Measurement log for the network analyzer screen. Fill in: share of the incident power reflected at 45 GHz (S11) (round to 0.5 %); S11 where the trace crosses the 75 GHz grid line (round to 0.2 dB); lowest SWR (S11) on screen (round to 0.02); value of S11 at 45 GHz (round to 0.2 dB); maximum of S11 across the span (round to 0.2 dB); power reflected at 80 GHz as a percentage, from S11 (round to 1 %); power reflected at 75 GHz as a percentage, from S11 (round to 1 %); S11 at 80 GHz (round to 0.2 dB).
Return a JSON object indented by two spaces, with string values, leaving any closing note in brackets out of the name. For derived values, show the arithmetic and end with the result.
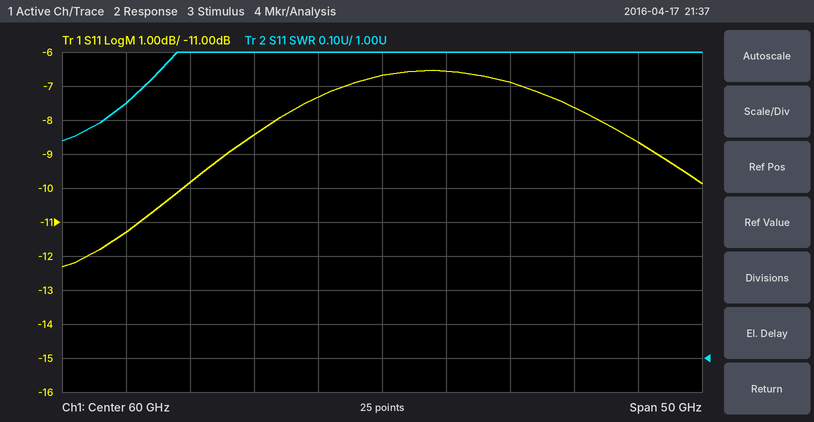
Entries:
{
  "share of the incident power reflected at 45 GHz (S11)": "10^(-9.8/10) ≈ 10.5 %",
  "S11 where the trace crosses the 75 GHz grid line": "-7.6 dB",
  "lowest SWR (S11) on screen": "1.64",
  "value of S11 at 45 GHz": "-9.8 dB",
  "maximum of S11 across the span": "-6.6 dB",
  "power reflected at 80 GHz as a percentage, from S11": "10^(-8.6/10) ≈ 14 %",
  "power reflected at 75 GHz as a percentage, from S11": "10^(-7.6/10) ≈ 17 %",
  "S11 at 80 GHz": "-8.6 dB"
}
